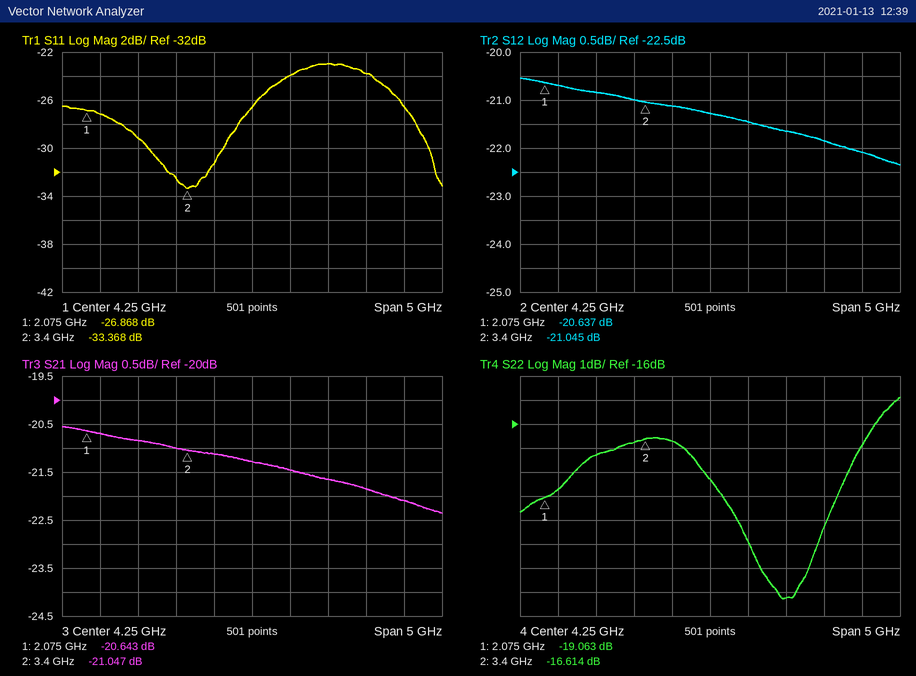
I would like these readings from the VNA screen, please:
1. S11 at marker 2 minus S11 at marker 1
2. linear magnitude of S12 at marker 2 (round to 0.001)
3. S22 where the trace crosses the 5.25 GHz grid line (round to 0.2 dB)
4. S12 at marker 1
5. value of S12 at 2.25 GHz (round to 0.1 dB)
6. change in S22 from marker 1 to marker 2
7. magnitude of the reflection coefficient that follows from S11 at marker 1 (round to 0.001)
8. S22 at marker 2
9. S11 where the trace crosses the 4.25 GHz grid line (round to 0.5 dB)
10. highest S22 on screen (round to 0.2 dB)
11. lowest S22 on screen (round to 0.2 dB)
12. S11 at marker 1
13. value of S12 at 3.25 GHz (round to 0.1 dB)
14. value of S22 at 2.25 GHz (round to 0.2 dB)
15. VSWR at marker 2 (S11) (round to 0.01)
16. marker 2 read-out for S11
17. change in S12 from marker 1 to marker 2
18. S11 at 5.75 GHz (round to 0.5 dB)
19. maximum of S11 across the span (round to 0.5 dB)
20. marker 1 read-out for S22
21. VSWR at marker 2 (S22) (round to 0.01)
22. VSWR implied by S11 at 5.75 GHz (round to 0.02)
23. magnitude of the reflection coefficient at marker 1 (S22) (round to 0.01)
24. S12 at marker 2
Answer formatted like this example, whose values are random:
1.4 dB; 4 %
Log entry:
-6.500 dB; 0.089; -23.2 dB; -20.637 dB; -20.7 dB; 2.449 dB; 0.045; -16.614 dB; -26.5 dB; -14.8 dB; -23.2 dB; -26.868 dB; -21.0 dB; -18.8 dB; 1.04; -33.368 dB; -0.408 dB; -24.0 dB; -23.0 dB; -19.063 dB; 1.35; 1.14; 0.11; -21.045 dB
